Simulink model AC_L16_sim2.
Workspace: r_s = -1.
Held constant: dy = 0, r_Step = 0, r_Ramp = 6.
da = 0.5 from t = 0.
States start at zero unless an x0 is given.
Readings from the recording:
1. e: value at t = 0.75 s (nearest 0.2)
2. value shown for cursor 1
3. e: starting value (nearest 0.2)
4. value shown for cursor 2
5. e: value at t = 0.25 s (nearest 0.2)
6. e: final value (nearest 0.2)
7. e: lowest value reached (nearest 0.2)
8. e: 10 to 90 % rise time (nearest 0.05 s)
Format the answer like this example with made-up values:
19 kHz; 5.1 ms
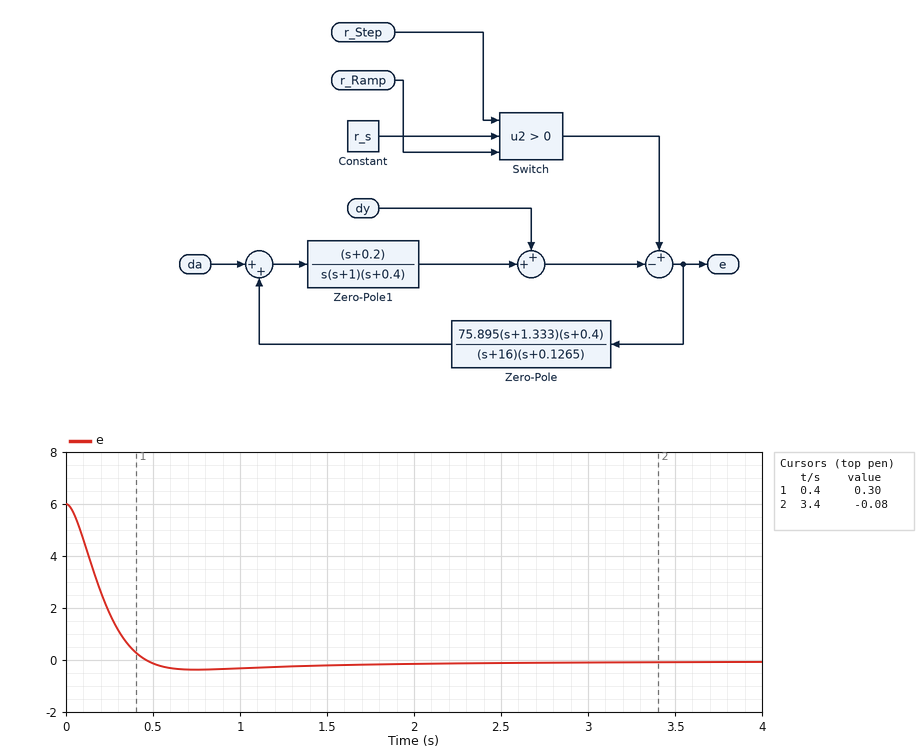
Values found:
-0.4; 0.30; 6.0; -0.08; 1.8; 0.0; -0.4; 0.30 s
